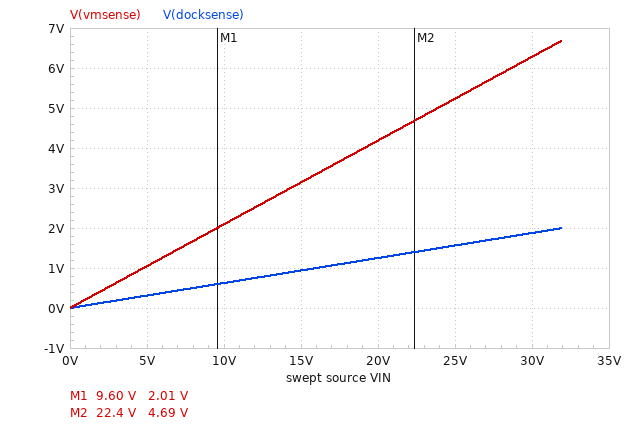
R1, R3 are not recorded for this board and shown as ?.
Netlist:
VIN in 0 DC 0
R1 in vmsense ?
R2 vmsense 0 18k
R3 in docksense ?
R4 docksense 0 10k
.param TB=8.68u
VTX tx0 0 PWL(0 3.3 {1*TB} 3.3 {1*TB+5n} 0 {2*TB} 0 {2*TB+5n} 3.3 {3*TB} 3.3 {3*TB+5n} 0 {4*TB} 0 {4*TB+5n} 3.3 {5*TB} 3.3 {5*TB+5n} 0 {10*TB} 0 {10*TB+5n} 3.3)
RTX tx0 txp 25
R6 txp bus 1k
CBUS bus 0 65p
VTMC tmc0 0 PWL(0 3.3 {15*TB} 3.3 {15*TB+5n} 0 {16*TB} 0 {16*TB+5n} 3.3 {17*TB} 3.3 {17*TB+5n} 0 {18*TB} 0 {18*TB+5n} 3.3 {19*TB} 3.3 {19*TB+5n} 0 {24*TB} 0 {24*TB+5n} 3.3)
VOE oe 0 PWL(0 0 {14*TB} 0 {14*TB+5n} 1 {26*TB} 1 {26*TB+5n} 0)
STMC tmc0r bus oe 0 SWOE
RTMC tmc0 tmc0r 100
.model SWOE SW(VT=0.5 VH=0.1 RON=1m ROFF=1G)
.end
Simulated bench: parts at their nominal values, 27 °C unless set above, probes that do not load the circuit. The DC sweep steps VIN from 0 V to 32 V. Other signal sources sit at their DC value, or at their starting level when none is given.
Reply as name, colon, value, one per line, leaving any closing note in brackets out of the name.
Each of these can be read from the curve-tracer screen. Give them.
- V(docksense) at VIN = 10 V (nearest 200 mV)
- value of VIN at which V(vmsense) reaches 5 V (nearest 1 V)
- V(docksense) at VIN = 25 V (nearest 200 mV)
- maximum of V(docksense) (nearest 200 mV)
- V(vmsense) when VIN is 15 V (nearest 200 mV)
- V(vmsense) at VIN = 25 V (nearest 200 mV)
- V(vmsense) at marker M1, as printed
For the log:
V(docksense) at VIN = 10 V: 600 mV
value of VIN at which V(vmsense) reaches 5 V: 24 V
V(docksense) at VIN = 25 V: 1.6 V
maximum of V(docksense): 2.0 V
V(vmsense) when VIN is 15 V: 3.2 V
V(vmsense) at VIN = 25 V: 5.2 V
V(vmsense) at marker M1, as printed: 2.01 V
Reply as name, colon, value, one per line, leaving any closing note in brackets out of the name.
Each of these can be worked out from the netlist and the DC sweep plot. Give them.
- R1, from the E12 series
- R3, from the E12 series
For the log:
R1, from the E12 series: 68 kΩ
R3, from the E12 series: 150 kΩ
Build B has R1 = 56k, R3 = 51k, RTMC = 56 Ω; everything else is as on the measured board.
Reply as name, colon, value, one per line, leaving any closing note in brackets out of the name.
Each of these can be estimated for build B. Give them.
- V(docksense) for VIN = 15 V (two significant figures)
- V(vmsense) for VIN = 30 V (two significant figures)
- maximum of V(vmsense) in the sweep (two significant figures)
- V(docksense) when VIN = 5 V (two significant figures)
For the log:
V(docksense) for VIN = 15 V: 2.5 V
V(vmsense) for VIN = 30 V: 7.3 V
maximum of V(vmsense) in the sweep: 7.8 V
V(docksense) when VIN = 5 V: 820 mV
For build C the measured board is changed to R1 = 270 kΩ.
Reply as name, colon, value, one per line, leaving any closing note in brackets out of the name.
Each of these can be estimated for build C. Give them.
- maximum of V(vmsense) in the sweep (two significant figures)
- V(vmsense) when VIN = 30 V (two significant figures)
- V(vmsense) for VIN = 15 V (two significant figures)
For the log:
maximum of V(vmsense) in the sweep: 2.0 V
V(vmsense) when VIN = 30 V: 1.9 V
V(vmsense) for VIN = 15 V: 940 mV
